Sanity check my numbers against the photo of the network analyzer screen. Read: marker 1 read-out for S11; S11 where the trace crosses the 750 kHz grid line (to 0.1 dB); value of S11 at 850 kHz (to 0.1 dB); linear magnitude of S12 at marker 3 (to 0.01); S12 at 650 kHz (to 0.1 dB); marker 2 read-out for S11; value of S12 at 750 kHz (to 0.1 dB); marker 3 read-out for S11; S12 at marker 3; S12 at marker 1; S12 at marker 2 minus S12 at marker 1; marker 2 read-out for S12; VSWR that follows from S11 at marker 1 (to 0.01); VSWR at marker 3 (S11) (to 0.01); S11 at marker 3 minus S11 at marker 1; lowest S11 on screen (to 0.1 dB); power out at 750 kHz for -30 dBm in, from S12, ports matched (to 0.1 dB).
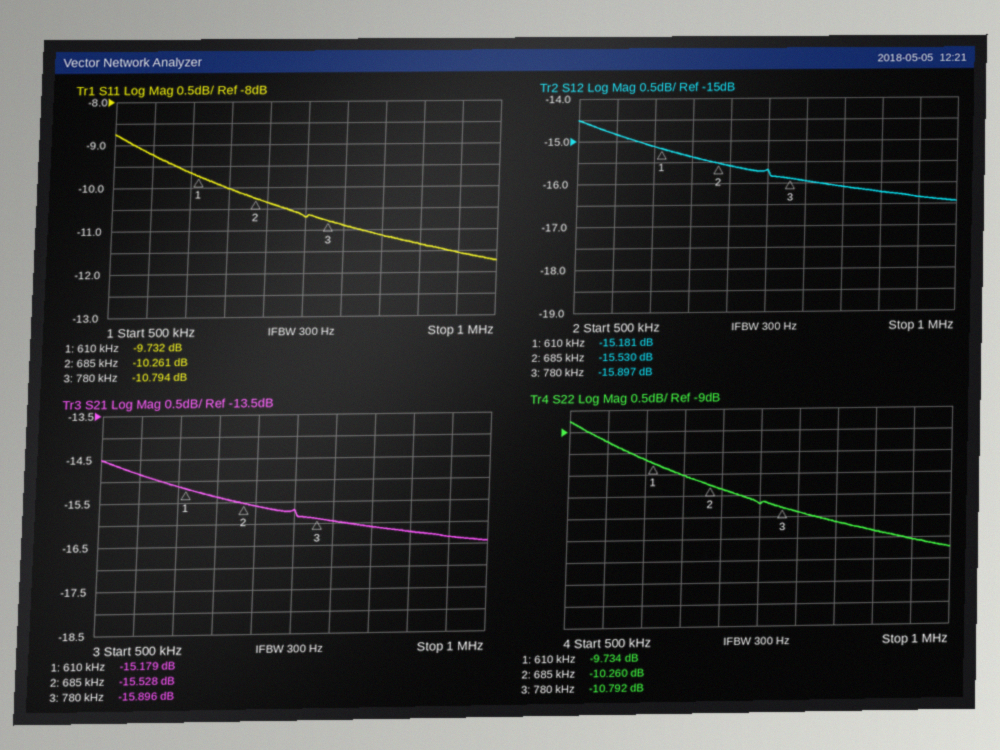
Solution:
-9.732 dB
-10.7 dB
-11.1 dB
0.16
-15.4 dB
-10.261 dB
-15.7 dB
-10.794 dB
-15.897 dB
-15.181 dB
-0.349 dB
-15.530 dB
1.97
1.81
-1.062 dB
-11.7 dB
-45.7 dBm
